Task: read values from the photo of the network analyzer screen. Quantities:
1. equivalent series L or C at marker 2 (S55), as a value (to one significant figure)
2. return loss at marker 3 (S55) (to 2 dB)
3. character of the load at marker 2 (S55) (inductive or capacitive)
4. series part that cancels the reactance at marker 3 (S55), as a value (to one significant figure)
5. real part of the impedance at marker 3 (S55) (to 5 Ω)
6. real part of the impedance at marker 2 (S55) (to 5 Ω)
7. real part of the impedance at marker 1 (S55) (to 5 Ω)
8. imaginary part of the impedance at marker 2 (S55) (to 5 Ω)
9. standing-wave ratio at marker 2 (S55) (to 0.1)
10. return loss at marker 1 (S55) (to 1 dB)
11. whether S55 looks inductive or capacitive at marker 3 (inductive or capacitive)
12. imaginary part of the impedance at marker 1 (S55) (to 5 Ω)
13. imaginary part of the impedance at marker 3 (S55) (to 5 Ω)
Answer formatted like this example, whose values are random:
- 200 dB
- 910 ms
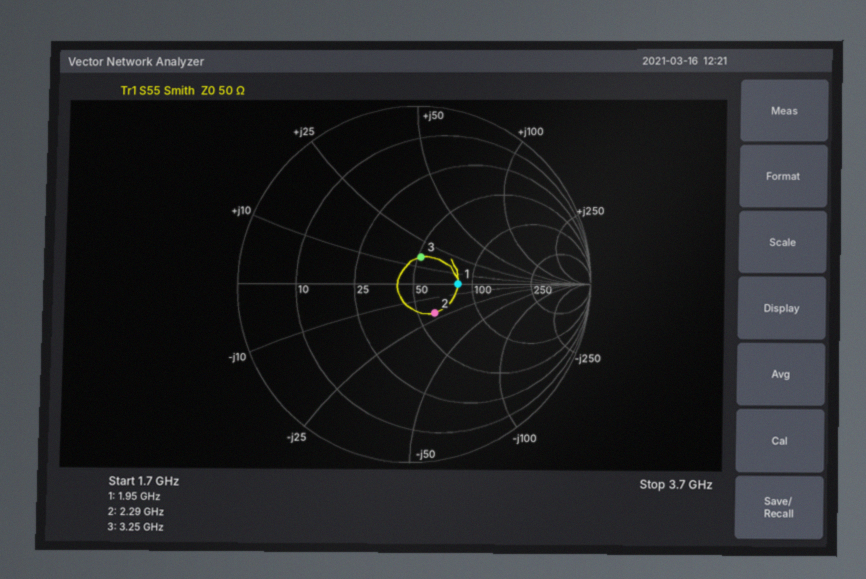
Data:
- 3 pF
- 16 dB
- capacitive
- 3 pF
- 50 Ω
- 60 Ω
- 85 Ω
- -20 Ω
- 1.5
- 12 dB
- inductive
- 0 Ω
- +15 Ω
